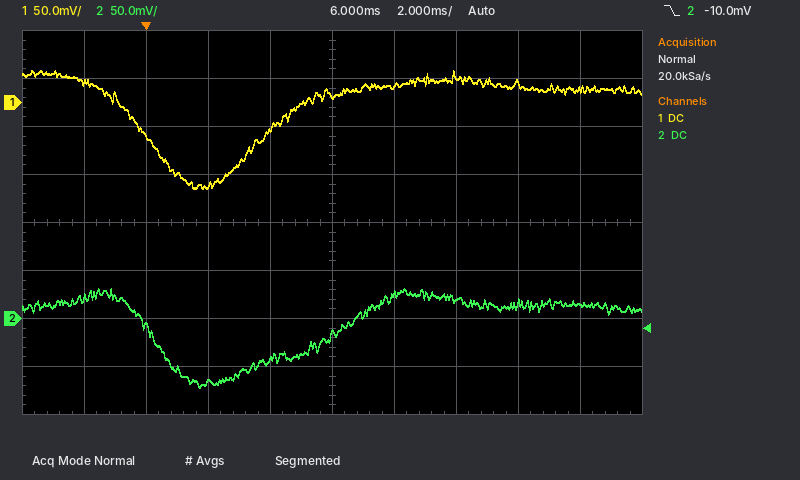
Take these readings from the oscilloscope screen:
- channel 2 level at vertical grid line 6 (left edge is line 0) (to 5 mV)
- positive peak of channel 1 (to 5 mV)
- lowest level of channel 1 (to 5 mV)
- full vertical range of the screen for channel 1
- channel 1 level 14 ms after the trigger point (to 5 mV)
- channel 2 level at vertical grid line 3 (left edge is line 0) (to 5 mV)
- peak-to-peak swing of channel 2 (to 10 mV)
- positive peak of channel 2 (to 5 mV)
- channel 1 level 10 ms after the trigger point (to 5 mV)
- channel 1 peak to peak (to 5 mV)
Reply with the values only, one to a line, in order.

25 mV
35 mV
-90 mV
400 mV
15 mV
-65 mV
100 mV
30 mV
30 mV
125 mV
